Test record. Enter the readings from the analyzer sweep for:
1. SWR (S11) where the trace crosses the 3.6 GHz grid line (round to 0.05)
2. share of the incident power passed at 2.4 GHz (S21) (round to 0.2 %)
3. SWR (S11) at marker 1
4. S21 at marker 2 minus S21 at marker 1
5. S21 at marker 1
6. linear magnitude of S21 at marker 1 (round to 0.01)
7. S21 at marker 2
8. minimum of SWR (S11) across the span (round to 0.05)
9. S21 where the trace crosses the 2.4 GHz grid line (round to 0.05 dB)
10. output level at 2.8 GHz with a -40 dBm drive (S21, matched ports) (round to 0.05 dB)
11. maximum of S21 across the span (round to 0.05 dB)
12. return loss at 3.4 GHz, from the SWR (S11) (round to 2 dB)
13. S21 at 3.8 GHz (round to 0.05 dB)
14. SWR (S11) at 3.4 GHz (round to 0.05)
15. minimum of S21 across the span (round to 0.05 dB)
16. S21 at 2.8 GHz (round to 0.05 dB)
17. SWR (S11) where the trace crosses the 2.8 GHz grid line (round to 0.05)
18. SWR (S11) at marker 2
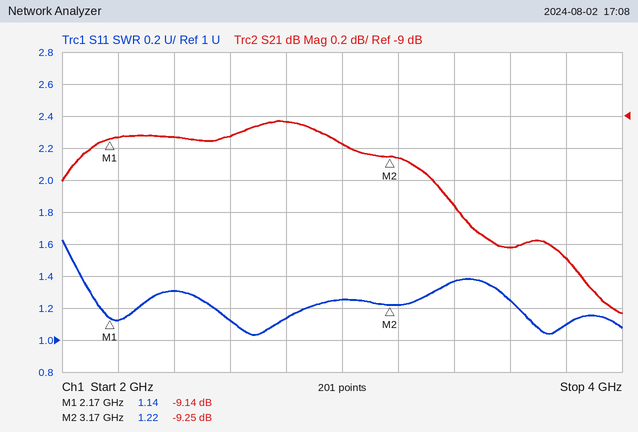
1.25
12.2 %
1.14
-0.11 dB
-9.14 dB
0.35
-9.25 dB
1.05
-9.15 dB
-49.05 dBm
-9.05 dB
16 dB
-9.90 dB
1.35
-10.25 dB
-9.05 dB
1.15
1.22
